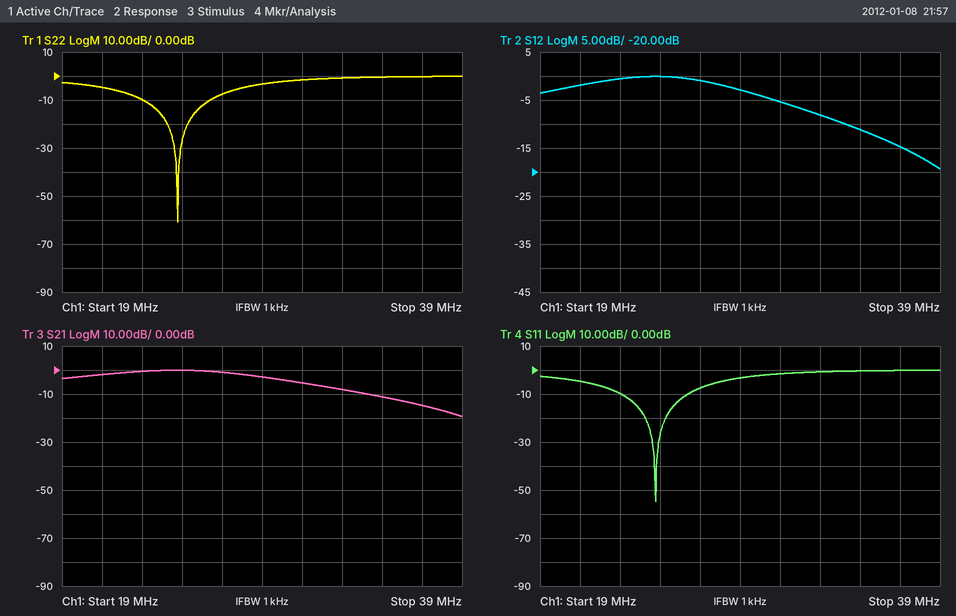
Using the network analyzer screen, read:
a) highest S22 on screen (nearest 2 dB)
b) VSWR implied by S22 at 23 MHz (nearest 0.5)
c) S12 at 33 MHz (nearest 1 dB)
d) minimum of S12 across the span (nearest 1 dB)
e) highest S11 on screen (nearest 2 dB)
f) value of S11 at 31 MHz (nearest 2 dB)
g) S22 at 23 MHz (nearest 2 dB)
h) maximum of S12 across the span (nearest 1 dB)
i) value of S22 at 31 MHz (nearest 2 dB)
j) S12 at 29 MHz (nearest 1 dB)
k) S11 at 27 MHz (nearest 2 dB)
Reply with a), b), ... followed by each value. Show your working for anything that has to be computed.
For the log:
a) 0 dB
b) |Γ| = 10^(-10/20) = 0.3162; VSWR = (1 + 0.3162)/(1 − 0.3162) ≈ 1.92, so 2.0 to the nearest 0.5
c) -8 dB
d) -19 dB
e) 0 dB
f) -2 dB
g) -10 dB
h) 0 dB
i) -2 dB
j) -3 dB
k) -8 dB
